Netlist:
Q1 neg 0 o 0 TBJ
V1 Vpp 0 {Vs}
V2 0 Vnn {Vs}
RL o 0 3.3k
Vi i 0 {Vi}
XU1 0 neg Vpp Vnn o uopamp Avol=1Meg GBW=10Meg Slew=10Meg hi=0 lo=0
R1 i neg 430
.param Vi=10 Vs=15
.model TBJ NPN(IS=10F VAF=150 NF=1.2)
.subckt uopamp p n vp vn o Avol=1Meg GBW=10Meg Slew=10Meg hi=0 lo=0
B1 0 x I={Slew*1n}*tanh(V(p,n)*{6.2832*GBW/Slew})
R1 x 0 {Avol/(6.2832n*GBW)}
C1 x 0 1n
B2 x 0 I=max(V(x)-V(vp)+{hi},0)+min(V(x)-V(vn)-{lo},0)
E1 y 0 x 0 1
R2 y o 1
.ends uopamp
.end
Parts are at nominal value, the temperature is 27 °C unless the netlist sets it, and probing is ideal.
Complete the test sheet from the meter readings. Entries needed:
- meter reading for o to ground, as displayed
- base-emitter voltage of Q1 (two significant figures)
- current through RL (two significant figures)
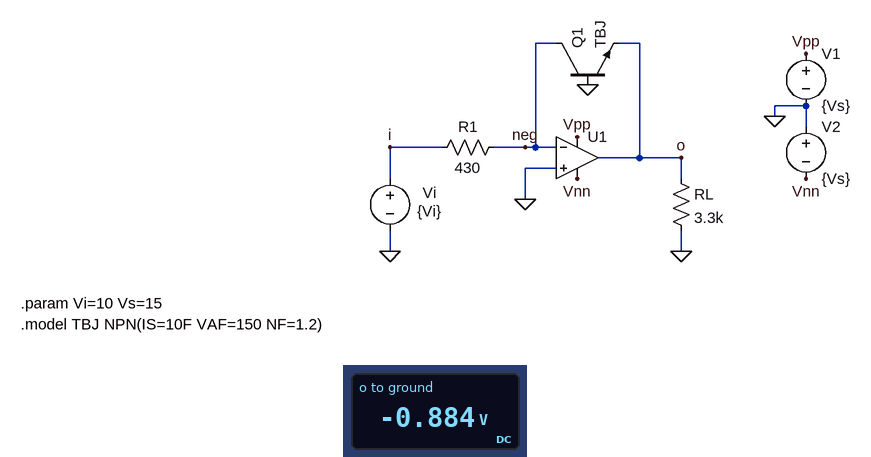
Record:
-0.884 V
880 mV
270 µA
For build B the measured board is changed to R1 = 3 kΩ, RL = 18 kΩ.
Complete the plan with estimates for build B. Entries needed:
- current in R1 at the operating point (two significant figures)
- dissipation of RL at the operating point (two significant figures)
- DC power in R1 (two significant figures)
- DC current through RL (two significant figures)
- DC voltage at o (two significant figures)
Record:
3.3 mA
38 µW
33 mW
46 µA
-820 mV
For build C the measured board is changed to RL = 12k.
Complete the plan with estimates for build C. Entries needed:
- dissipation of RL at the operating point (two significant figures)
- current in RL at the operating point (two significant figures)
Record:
65 µW
74 µA
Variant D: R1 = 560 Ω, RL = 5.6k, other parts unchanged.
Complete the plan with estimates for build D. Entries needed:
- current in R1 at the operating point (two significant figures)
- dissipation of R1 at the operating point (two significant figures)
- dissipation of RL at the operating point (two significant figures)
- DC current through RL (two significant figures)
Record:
18 mA
180 mW
140 µW
160 µA
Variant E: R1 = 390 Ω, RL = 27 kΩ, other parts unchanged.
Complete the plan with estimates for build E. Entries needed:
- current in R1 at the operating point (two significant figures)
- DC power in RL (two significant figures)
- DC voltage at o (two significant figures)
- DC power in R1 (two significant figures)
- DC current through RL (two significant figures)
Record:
26 mA
29 µW
-890 mV
260 mW
33 µA
